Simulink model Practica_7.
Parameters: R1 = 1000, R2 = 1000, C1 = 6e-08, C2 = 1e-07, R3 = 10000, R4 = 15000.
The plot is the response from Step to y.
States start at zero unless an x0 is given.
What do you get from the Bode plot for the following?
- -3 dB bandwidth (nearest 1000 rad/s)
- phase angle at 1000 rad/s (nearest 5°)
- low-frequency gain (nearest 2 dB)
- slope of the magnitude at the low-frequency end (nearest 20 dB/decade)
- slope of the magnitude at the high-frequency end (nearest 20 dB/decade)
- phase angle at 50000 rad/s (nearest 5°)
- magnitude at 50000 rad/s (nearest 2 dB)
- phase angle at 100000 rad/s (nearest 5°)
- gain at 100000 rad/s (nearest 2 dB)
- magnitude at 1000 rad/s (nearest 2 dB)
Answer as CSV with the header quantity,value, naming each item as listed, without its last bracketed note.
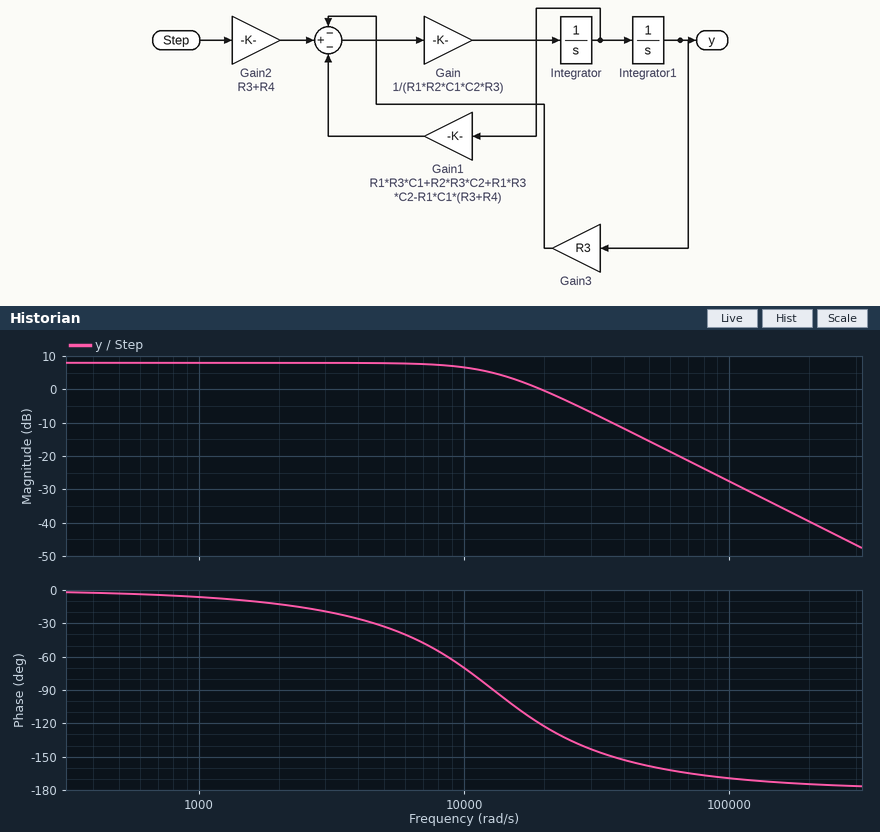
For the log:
quantity,value
-3 dB bandwidth,13000 rad/s
phase angle at 1000 rad/s,-5°
low-frequency gain,8 dB
slope of the magnitude at the low-frequency end,0 dB/decade
slope of the magnitude at the high-frequency end,-40 dB/decade
phase angle at 50000 rad/s,-160°
magnitude at 50000 rad/s,-16 dB
phase angle at 100000 rad/s,-170°
gain at 100000 rad/s,-28 dB
magnitude at 1000 rad/s,8 dB
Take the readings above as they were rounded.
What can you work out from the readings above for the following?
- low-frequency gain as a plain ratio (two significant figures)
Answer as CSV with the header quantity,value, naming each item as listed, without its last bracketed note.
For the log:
quantity,value
low-frequency gain as a plain ratio,2.5
